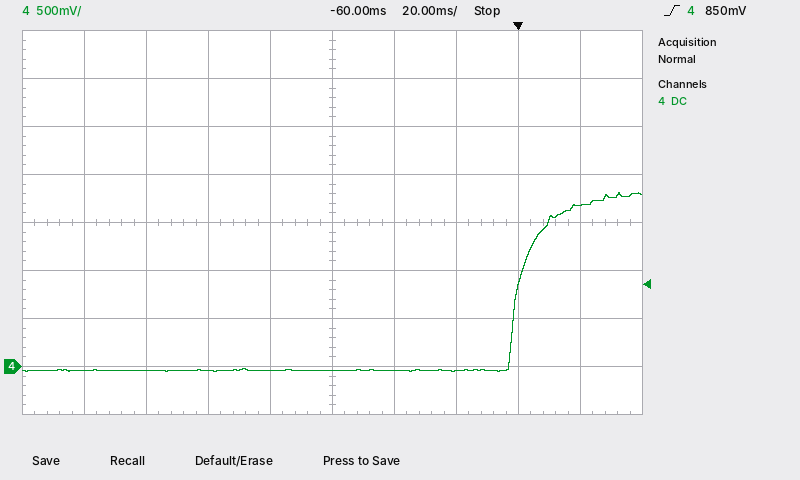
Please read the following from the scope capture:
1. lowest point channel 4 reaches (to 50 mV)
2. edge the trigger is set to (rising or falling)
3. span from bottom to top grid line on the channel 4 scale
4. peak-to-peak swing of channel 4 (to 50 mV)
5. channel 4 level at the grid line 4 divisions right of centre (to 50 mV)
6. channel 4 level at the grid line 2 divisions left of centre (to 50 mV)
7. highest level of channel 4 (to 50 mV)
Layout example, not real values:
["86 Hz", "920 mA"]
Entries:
["-50 mV", "rising", "4 V", "1.85 V", "1.70 V", "-50 mV", "1.80 V"]
